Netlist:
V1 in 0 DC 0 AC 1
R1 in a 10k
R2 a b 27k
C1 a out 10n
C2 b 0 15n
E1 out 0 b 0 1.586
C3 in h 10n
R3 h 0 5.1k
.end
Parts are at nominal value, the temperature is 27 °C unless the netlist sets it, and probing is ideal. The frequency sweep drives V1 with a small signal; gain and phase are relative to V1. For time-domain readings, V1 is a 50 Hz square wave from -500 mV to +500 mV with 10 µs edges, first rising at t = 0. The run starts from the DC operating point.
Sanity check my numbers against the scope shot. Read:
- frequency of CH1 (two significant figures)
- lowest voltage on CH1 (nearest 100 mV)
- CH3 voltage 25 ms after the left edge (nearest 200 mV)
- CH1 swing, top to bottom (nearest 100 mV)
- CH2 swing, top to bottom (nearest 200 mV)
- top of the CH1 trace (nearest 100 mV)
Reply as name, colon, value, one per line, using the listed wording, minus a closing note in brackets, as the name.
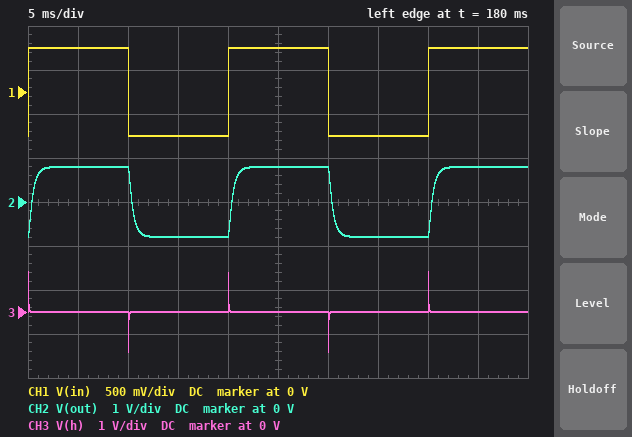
frequency of CH1: 50 Hz
lowest voltage on CH1: -500 mV
CH3 voltage 25 ms after the left edge: 0 V
CH1 swing, top to bottom: 1.0 V
CH2 swing, top to bottom: 1.6 V
top of the CH1 trace: 500 mV
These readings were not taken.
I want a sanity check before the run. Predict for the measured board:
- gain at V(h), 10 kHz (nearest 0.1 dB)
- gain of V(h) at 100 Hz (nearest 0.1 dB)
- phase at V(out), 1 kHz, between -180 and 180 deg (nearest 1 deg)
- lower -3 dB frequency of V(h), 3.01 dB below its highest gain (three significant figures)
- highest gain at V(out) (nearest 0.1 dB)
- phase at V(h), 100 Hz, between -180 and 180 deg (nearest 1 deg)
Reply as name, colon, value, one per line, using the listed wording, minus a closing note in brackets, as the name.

gain at V(h), 10 kHz: -0.4 dB
gain of V(h) at 100 Hz: -29.9 dB
phase at V(out), 1 kHz, between -180 and 180 deg: -101 deg
lower -3 dB frequency of V(h), 3.01 dB below its highest gain: 3.12 kHz
highest gain at V(out): 4.0 dB
phase at V(h), 100 Hz, between -180 and 180 deg: 88 deg
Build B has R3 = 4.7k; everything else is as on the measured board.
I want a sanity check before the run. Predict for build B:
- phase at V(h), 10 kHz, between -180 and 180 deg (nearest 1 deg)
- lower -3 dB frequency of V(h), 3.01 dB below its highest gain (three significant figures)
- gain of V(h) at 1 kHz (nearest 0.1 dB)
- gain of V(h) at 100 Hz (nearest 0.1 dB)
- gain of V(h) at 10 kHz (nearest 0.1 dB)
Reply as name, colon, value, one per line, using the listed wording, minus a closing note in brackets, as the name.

phase at V(h), 10 kHz, between -180 and 180 deg: 19 deg
lower -3 dB frequency of V(h), 3.01 dB below its highest gain: 3.39 kHz
gain of V(h) at 1 kHz: -11.0 dB
gain of V(h) at 100 Hz: -30.6 dB
gain of V(h) at 10 kHz: -0.5 dB
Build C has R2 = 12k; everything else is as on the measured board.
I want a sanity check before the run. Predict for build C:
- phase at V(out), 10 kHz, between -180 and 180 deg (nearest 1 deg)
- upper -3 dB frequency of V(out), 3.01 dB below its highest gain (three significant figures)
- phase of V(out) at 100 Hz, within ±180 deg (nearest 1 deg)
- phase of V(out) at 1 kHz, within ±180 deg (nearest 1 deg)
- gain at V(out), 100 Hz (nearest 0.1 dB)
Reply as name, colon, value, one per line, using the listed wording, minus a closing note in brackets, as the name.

phase at V(out), 10 kHz, between -180 and 180 deg: -166 deg
upper -3 dB frequency of V(out), 3.01 dB below its highest gain: 751 Hz
phase of V(out) at 100 Hz, within ±180 deg: -10 deg
phase of V(out) at 1 kHz, within ±180 deg: -80 deg
gain at V(out), 100 Hz: 3.9 dB
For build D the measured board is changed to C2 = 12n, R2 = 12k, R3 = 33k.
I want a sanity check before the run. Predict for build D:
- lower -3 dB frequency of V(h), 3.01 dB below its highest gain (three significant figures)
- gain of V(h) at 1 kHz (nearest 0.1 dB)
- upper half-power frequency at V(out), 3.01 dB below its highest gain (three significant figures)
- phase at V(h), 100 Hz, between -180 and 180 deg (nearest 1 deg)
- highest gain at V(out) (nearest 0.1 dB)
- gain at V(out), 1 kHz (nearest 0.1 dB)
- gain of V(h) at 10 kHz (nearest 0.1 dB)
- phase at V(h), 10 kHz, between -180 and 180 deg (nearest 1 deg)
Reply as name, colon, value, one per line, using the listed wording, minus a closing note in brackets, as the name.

lower -3 dB frequency of V(h), 3.01 dB below its highest gain: 482 Hz
gain of V(h) at 1 kHz: -0.9 dB
upper half-power frequency at V(out), 3.01 dB below its highest gain: 1.06 kHz
phase at V(h), 100 Hz, between -180 and 180 deg: 78 deg
highest gain at V(out): 4.0 dB
gain at V(out), 1 kHz: 1.3 dB
gain of V(h) at 10 kHz: 0 dB
phase at V(h), 10 kHz, between -180 and 180 deg: 3 deg
